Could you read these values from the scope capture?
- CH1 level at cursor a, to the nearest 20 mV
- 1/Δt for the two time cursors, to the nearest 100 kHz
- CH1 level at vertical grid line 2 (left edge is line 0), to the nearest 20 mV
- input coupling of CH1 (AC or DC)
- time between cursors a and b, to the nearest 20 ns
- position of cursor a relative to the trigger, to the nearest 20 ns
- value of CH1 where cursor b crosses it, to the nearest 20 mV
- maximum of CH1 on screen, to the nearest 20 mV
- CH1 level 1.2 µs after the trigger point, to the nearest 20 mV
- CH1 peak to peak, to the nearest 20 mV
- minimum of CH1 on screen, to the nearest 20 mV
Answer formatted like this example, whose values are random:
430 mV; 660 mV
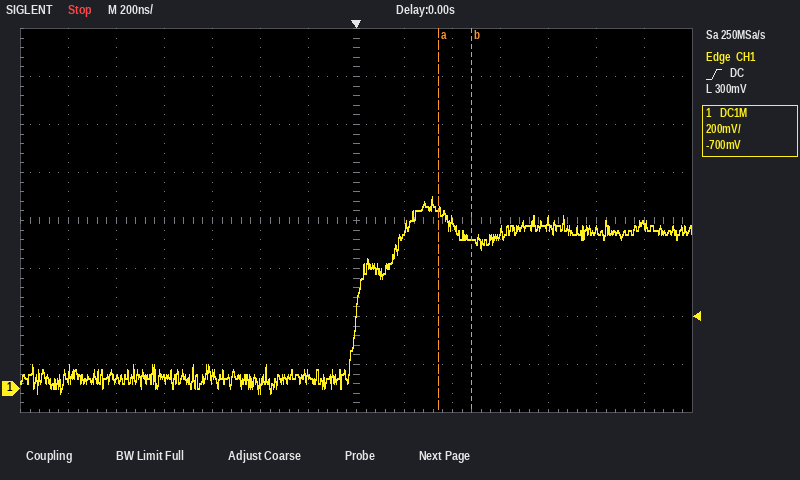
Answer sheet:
740 mV; 7.1 MHz; 40 mV; DC; 140 ns; +340 ns; 620 mV; 800 mV; 680 mV; 820 mV; -20 mV
